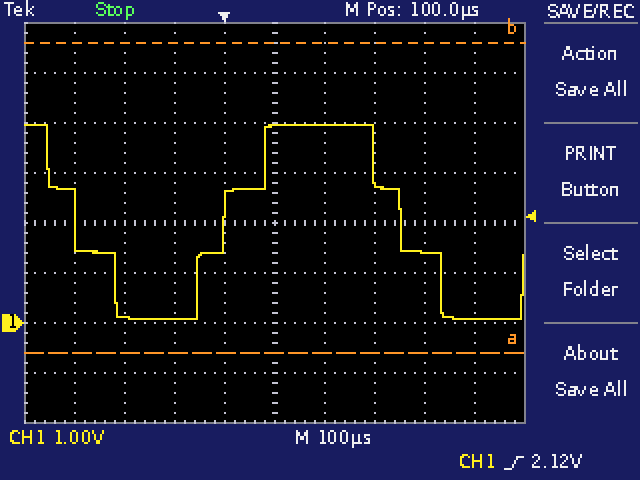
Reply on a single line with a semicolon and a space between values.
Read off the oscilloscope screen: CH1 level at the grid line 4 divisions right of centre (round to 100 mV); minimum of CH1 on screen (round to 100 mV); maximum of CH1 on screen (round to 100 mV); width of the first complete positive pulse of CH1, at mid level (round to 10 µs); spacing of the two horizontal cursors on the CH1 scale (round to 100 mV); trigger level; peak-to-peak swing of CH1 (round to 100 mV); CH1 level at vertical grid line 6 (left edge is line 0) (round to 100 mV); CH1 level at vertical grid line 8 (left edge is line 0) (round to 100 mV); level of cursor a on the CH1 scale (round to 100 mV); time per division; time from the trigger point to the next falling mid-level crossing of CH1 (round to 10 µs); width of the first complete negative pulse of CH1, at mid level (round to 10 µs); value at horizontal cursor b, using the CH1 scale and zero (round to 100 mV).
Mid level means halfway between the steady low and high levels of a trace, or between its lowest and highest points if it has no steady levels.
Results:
100 mV; 100 mV; 4.0 V; 350 µs; 6.2 V; 2.12 V; 3.9 V; 4.0 V; 1.4 V; -600 mV; 100 µs; 350 µs; 300 µs; 5.6 V
